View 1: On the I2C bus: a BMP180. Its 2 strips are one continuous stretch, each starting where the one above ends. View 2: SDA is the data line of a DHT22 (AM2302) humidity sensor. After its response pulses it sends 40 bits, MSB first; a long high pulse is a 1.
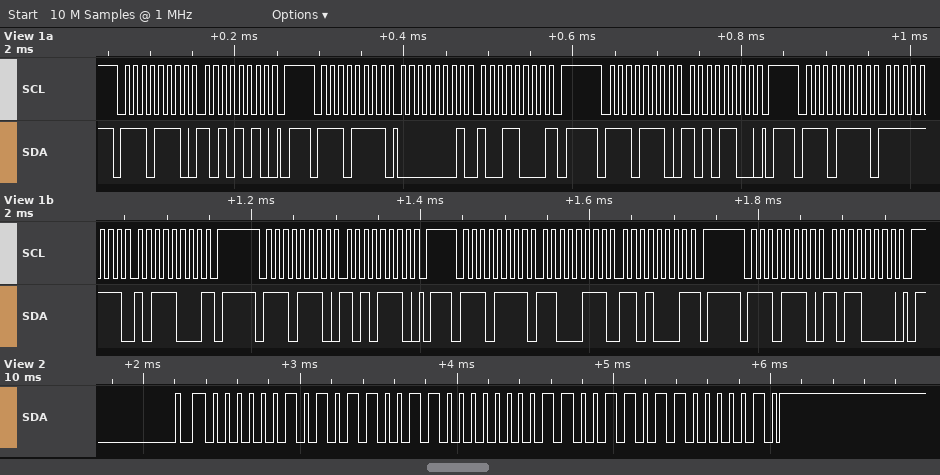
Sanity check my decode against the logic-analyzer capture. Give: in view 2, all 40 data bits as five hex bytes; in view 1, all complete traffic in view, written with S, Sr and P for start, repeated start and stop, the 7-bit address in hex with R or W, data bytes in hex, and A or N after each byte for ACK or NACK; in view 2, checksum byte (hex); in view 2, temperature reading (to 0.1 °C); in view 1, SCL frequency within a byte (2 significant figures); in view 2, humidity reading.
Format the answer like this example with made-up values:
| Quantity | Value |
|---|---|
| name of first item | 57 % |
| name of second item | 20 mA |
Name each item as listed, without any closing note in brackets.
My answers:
| Quantity | Value |
|---|---|
| in view 2, all 40 data bits as five hex bytes | 02 B3 00 CD 82 |
| in view 1, all complete traffic in view, written with S, Sr and P for start, repeated start and stop, the 7-bit address in hex with R or W, data bytes in hex, and A or N after each byte for ACK or NACK | S 77W A AA A P S 77R A 01 A 98 N P S 77W A AC A P S 77R A FF A B8 N P S 77W A AE A P S 77R A C7 A D1 N P S 77W A B0 A P |
| in view 2, checksum byte | 0x82 |
| in view 2, temperature reading | 20.5 °C |
| in view 1, SCL frequency within a byte | 100 kHz |
| in view 2, humidity reading | 69.1 % |
